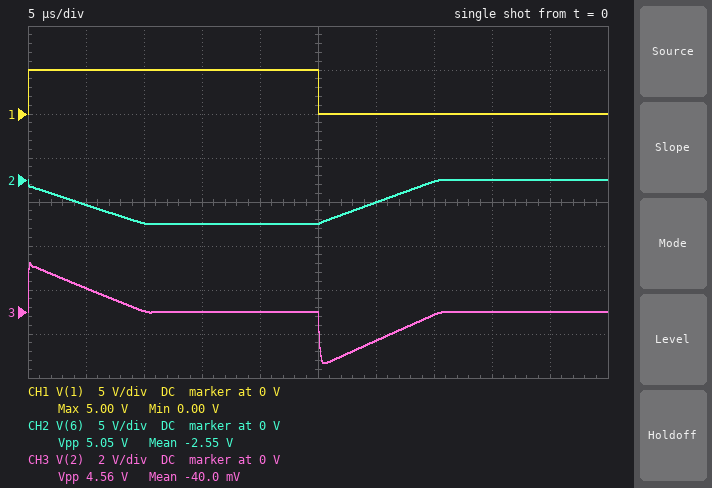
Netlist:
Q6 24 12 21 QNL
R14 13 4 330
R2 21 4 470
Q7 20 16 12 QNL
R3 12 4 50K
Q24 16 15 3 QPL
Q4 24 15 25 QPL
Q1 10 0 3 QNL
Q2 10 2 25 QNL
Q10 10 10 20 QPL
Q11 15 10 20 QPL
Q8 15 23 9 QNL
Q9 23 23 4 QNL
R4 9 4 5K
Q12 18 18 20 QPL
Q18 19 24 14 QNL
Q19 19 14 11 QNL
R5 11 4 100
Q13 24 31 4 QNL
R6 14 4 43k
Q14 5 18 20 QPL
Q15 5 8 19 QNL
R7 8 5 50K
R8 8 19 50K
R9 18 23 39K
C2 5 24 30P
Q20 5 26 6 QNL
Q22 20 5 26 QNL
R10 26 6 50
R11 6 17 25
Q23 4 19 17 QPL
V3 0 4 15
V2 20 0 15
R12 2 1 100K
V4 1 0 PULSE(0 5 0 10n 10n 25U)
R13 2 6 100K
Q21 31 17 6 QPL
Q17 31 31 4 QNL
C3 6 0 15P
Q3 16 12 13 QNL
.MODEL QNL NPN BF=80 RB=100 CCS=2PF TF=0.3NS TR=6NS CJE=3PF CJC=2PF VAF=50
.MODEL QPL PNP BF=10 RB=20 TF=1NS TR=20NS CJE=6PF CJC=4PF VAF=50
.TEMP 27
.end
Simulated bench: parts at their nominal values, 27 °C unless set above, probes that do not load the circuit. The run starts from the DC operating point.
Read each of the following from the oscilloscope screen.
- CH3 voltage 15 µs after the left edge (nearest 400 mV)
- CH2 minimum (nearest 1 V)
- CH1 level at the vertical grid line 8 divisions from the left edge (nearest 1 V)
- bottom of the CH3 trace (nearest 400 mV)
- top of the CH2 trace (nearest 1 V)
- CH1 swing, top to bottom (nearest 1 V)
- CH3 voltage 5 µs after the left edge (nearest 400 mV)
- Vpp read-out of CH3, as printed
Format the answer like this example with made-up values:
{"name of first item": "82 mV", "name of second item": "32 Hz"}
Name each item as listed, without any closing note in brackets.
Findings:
{"CH3 voltage 15 µs after the left edge": "0 V", "CH2 minimum": "-5 V", "CH1 level at the vertical grid line 8 divisions from the left edge": "0 V", "bottom of the CH3 trace": "-2.4 V", "top of the CH2 trace": "0 V", "CH1 swing, top to bottom": "5 V", "CH3 voltage 5 µs after the left edge": "1.2 V", "Vpp read-out of CH3, as printed": "4.56 V"}
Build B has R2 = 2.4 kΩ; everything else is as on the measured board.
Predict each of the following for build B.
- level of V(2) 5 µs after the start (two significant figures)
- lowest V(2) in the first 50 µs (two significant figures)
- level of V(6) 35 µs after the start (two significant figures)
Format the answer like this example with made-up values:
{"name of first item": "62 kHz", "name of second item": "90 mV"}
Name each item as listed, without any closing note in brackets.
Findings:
{"level of V(2) 5 µs after the start": "1.0 V", "lowest V(2) in the first 50 µs": "-2.4 V", "level of V(6) 35 µs after the start": "-2.2 V"}
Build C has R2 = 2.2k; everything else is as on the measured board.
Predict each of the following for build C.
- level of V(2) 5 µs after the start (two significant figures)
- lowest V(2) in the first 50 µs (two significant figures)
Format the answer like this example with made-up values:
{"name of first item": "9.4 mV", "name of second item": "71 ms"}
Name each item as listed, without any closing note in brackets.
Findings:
{"level of V(2) 5 µs after the start": "1.0 V", "lowest V(2) in the first 50 µs": "-2.4 V"}
